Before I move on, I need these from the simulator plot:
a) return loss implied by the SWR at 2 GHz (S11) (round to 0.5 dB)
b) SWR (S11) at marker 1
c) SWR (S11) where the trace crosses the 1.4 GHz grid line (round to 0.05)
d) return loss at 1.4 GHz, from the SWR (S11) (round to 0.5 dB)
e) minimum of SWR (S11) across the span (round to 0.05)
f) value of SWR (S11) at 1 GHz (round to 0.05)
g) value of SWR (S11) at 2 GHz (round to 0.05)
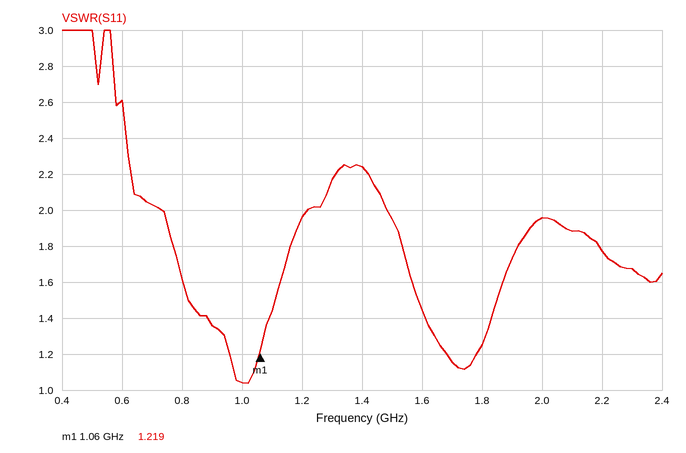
10.0 dB
1.219
2.25
8.5 dB
1.05
1.05
1.95
